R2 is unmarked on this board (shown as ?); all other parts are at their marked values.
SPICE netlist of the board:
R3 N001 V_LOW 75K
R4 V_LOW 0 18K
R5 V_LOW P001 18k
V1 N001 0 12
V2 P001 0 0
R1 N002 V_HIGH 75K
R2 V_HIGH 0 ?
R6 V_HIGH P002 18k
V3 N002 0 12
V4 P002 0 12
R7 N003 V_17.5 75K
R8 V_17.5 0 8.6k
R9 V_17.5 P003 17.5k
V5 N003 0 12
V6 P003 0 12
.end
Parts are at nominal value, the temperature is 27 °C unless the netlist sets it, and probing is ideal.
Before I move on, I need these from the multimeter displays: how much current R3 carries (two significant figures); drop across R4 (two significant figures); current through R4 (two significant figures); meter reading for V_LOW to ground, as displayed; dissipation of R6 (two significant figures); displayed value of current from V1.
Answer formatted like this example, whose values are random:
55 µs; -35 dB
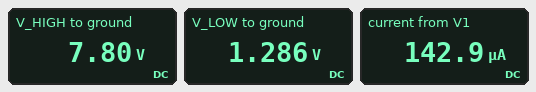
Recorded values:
140 µA; 1.3 V; 71 µA; 1.286 V; 980 µW; 142.9 µA
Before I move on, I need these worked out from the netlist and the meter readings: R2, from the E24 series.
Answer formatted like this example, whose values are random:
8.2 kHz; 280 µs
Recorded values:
27 kΩ
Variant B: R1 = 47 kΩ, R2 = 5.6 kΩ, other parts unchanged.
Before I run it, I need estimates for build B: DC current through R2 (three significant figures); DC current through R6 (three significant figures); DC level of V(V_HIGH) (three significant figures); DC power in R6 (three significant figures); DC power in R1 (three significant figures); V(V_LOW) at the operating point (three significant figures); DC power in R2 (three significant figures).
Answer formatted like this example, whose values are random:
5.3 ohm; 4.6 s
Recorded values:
645 µA; 466 µA; 3.61 V; 3.91 mW; 1.50 mW; 1.29 V; 2.33 mW
